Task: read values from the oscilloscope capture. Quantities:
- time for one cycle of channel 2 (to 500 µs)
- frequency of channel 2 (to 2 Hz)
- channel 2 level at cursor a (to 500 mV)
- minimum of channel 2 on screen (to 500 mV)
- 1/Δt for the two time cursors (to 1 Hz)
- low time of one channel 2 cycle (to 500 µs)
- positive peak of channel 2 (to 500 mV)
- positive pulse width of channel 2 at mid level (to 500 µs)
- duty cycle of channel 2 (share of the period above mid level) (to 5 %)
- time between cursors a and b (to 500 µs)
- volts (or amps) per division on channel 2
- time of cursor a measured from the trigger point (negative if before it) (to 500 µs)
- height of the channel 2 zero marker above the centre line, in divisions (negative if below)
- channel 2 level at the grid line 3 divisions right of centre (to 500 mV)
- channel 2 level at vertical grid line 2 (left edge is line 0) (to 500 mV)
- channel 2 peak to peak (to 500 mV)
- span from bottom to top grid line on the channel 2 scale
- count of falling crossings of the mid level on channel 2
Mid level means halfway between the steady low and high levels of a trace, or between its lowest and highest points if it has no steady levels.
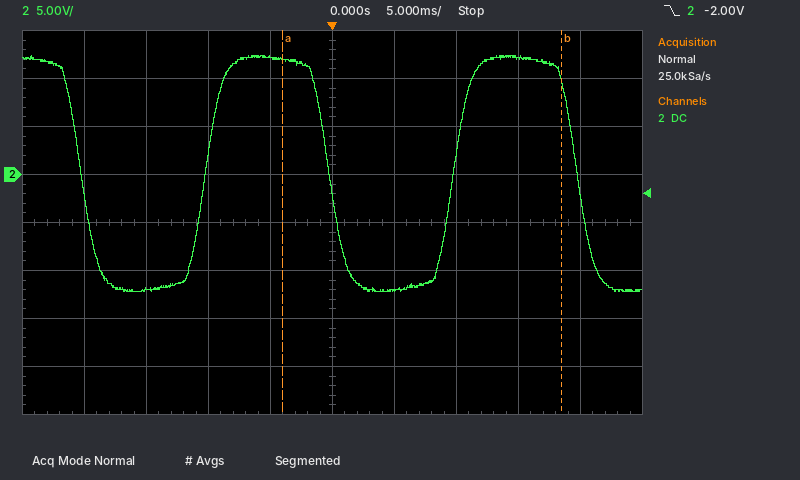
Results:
20.0 ms
50 Hz
12.0 V
-12.0 V
44 Hz
10.0 ms
12.5 V
10.0 ms
50 %
22.5 ms
5 V
-4.0 ms
+1.0 div
12.0 V
-12.0 V
24.5 V
40 V
3
